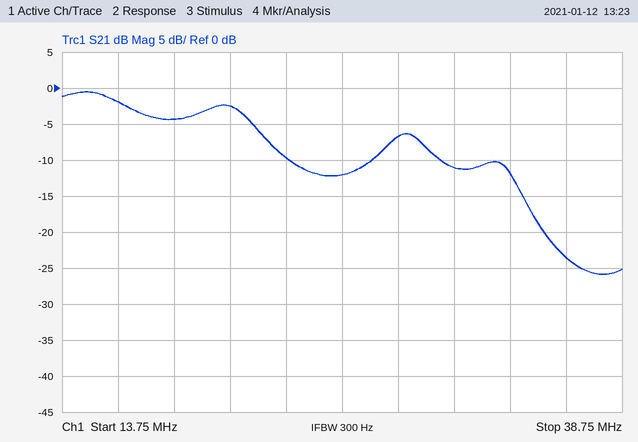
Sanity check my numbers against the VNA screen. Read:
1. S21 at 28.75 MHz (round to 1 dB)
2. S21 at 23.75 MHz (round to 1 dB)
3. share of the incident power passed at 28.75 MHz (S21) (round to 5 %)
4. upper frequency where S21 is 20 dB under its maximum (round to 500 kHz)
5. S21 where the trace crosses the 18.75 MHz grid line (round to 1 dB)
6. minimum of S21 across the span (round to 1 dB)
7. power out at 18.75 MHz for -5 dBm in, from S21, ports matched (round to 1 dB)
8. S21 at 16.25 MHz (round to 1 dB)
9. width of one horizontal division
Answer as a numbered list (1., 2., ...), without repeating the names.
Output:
1. -7 dB
2. -10 dB
3. 20 %
4. 35.5 MHz
5. -4 dB
6. -26 dB
7. -9 dBm
8. -2 dB
9. 2.5 MHz
